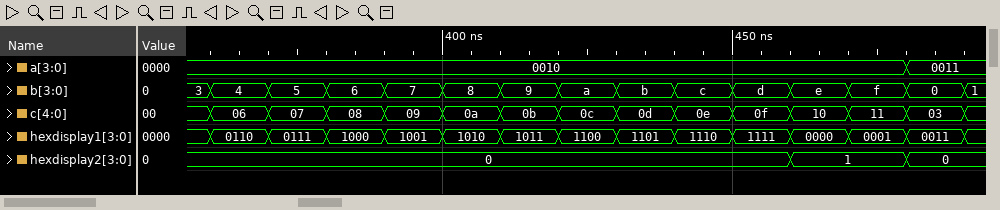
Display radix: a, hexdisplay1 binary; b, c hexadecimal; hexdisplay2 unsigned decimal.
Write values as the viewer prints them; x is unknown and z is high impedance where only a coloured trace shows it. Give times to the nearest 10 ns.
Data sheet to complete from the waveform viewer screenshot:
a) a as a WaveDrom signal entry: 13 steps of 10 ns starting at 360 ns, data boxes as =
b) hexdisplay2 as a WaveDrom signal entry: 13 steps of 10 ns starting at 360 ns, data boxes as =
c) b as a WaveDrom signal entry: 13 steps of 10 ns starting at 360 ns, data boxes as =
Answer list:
{name: 'a', wave: '=...........=', data: '0010 0011'}
{name: 'hexdisplay2', wave: '=.........=.=', data: '0 1 0'}
{name: 'b', wave: '=============', data: '4 5 6 7 8 9 a b c d e f 0'}
